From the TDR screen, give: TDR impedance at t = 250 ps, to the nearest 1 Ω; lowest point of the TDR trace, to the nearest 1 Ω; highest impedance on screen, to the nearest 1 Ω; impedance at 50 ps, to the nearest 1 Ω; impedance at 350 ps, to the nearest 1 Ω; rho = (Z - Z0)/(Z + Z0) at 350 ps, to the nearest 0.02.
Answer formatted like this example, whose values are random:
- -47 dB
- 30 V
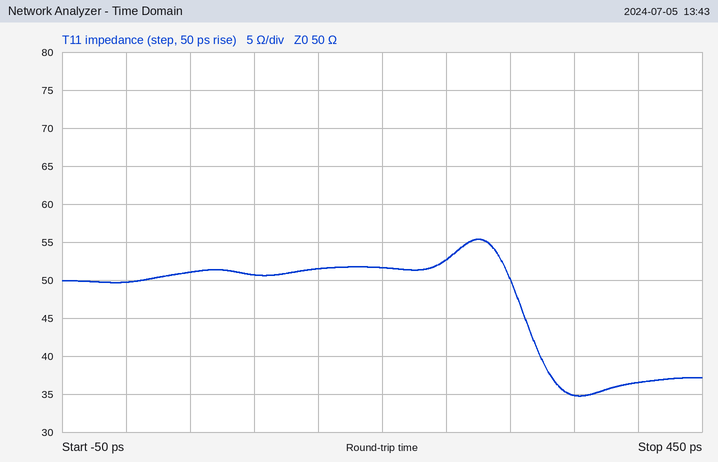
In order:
- 53 Ω
- 35 Ω
- 55 Ω
- 51 Ω
- 35 Ω
- -0.18
